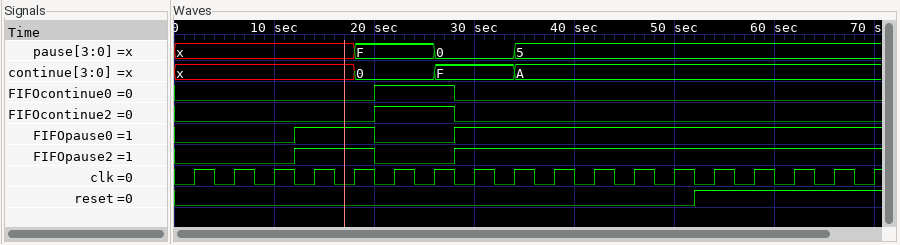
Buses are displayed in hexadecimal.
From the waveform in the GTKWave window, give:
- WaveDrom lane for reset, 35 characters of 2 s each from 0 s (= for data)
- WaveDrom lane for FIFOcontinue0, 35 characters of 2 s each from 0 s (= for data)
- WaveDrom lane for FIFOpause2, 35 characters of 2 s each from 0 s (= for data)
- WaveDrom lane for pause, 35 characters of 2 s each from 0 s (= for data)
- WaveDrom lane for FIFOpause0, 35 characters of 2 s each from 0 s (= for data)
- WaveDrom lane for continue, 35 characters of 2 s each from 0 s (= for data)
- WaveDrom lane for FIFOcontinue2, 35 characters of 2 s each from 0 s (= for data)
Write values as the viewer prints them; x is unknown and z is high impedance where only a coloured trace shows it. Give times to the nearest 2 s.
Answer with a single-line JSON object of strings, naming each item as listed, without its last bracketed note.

{"WaveDrom lane for reset, 35 characters of 2 s each from 0 s": "{name: 'reset', wave: '0.........................1........'}", "WaveDrom lane for FIFOcontinue0, 35 characters of 2 s each from 0 s": "{name: 'FIFOcontinue0', wave: '0.........1...0....................'}", "WaveDrom lane for FIFOpause2, 35 characters of 2 s each from 0 s": "{name: 'FIFOpause2', wave: '0.....1...0...1....................'}", "WaveDrom lane for pause, 35 characters of 2 s each from 0 s": "{name: 'pause', wave: 'x........=...=...=.................', data: 'F 0 5'}", "WaveDrom lane for FIFOpause0, 35 characters of 2 s each from 0 s": "{name: 'FIFOpause0', wave: '0.....1...0...1....................'}", "WaveDrom lane for continue, 35 characters of 2 s each from 0 s": "{name: 'continue', wave: 'x........=...=...=.................', data: '0 F A'}", "WaveDrom lane for FIFOcontinue2, 35 characters of 2 s each from 0 s": "{name: 'FIFOcontinue2', wave: '0.........1...0....................'}"}
